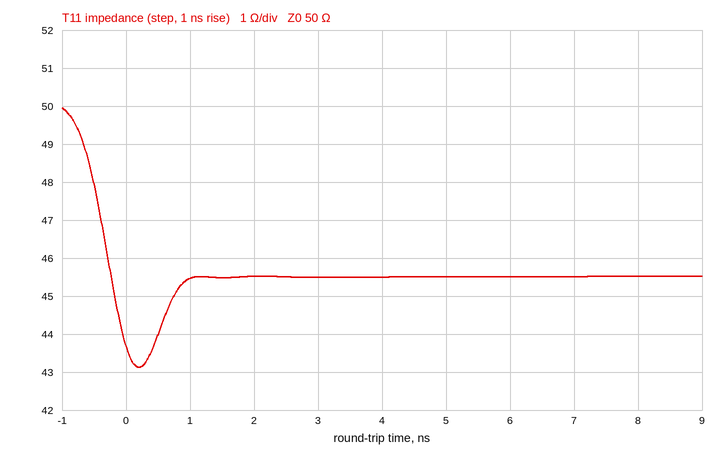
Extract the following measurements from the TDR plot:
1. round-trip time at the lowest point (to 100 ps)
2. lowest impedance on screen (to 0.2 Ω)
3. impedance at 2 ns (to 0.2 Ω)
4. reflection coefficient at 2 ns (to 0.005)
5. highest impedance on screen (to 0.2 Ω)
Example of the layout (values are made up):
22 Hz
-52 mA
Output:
200 ps
43.2 Ω
45.6 Ω
-0.045
50.0 Ω
